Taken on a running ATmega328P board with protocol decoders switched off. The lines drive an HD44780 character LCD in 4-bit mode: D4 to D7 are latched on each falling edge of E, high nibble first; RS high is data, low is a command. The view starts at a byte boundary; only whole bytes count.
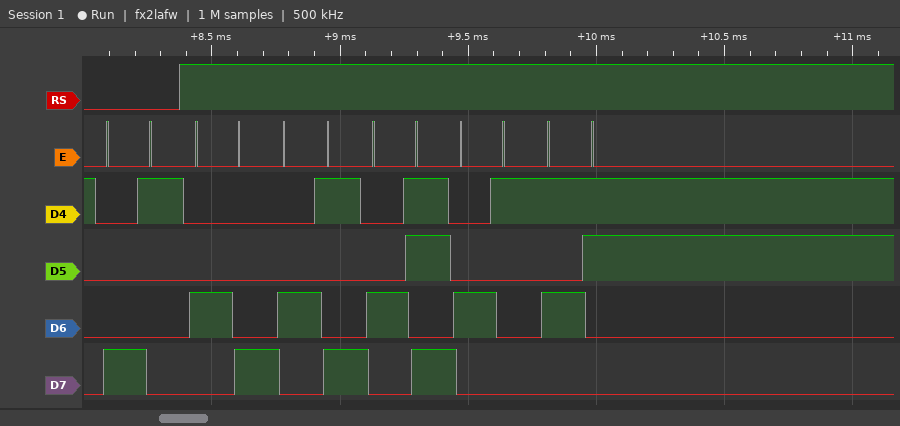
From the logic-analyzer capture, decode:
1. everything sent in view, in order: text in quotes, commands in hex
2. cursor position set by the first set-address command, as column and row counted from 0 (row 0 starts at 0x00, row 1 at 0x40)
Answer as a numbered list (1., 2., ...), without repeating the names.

1. 0x81 "HIKAS"
2. column 1, row 0
